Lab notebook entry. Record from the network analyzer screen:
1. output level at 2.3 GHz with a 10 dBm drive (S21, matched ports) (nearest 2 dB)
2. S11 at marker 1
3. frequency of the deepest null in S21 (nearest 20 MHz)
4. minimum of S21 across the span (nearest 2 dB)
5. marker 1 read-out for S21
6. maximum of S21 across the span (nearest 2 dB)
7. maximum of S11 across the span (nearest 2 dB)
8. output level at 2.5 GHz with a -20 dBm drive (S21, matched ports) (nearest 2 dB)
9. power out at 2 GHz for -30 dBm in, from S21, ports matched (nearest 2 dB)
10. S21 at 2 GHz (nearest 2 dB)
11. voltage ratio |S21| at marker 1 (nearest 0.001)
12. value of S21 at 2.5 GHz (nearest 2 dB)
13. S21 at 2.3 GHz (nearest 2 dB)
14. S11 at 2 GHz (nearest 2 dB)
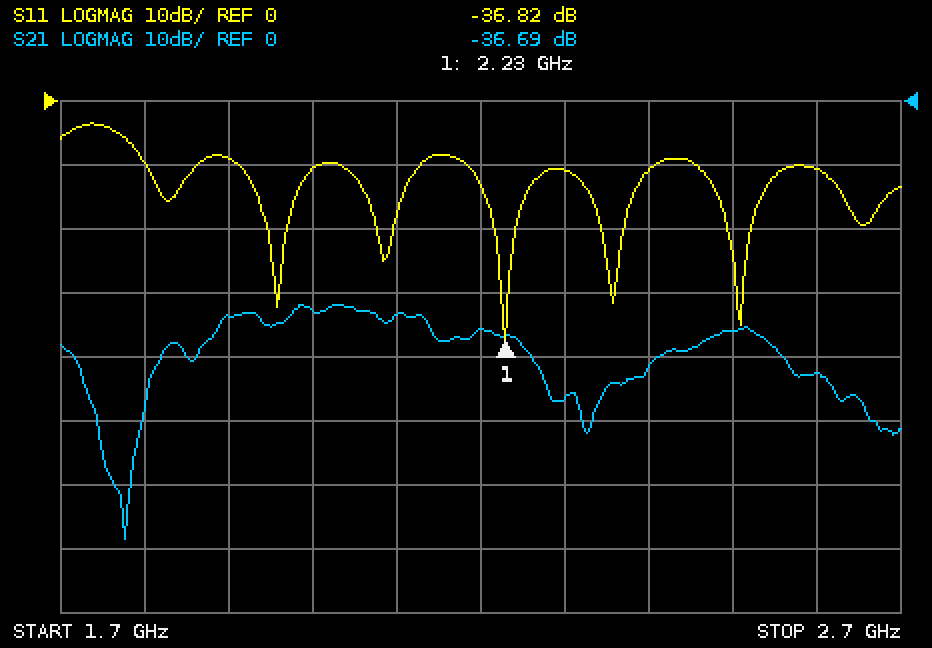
-36 dBm
-36.82 dB
1.78 GHz
-68 dB
-36.69 dB
-32 dB
-4 dB
-56 dBm
-62 dBm
-32 dB
0.015
-36 dB
-46 dB
-10 dB
